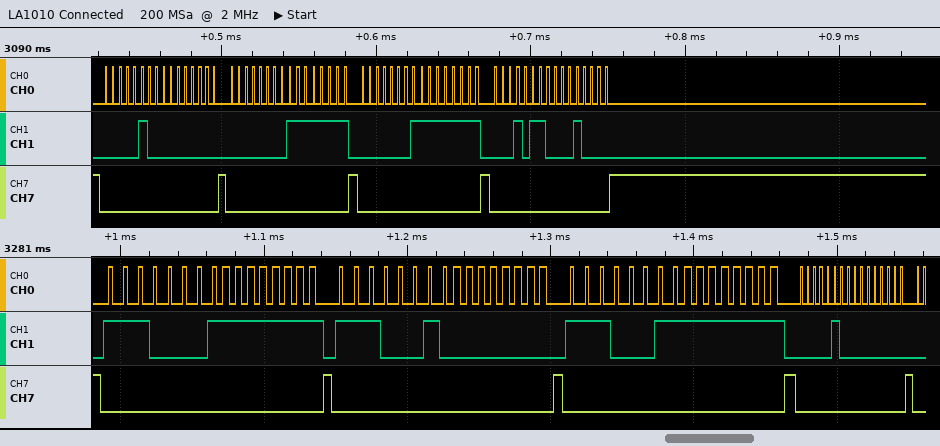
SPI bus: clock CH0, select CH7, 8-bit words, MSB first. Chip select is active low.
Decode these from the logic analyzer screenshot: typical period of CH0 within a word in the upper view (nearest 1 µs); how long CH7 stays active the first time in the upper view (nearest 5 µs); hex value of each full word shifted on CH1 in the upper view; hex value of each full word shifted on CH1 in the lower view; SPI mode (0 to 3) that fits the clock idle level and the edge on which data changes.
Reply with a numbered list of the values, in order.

1. 5 µs
2. 75 µs
3. 04, 00, 00, FF, 01, FF, 16, 10
4. E1, FF, E2, 00, E3, FF, 04, 00
5. 1
